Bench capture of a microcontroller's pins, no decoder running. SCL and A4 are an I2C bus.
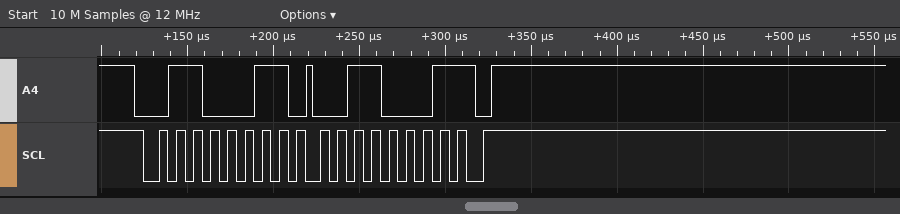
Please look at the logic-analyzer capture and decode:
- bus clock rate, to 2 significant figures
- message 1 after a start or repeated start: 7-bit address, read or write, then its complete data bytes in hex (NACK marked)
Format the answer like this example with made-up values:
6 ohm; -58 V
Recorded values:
100 kHz; 0x31 read: 31 NACK
